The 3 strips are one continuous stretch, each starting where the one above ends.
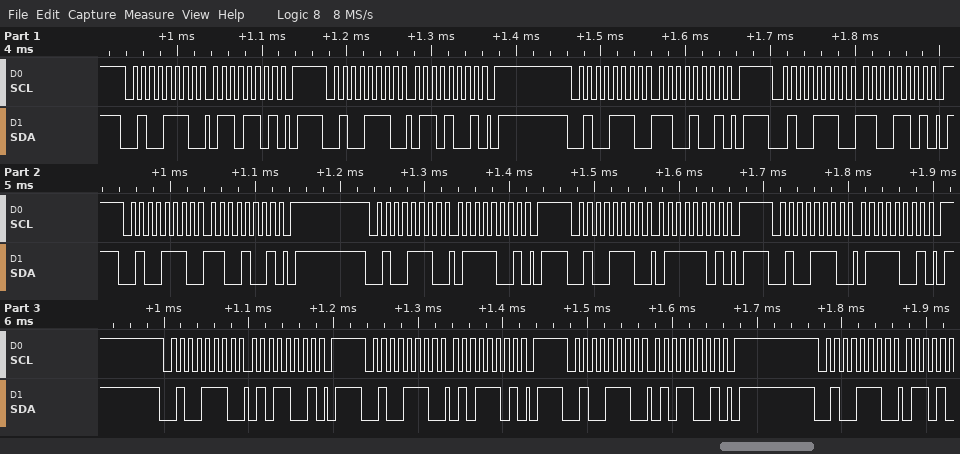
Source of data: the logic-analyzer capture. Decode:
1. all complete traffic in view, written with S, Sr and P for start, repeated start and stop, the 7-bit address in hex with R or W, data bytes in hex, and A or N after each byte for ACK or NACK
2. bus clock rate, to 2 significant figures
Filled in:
S 27W A 6D A P S 27W A 69 A P S 27W A C9 A P S 27W A CD A P S 27W A C9 A P S 27W A 79 A P S 27W A 7D A P S 27W A 79 A P S 27W A 59 A P S 27W A 5D A P S 27W A 59 A P S 27W A
100 kHz
